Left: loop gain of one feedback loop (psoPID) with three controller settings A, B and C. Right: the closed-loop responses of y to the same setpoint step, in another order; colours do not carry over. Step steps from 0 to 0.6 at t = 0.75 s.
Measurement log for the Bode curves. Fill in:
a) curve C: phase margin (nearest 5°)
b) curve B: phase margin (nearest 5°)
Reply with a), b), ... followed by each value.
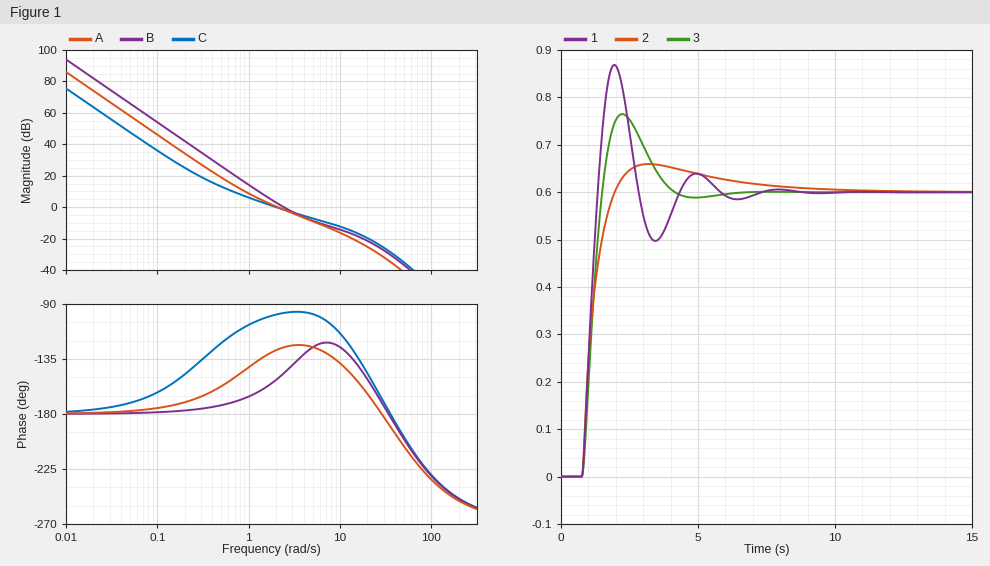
a) 80°
b) 35°
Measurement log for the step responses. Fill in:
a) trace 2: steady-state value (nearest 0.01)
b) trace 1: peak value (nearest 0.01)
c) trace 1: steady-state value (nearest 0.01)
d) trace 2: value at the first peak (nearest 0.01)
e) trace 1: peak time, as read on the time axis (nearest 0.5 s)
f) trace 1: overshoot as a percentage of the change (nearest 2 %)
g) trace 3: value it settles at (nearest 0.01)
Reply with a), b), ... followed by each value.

a) 0.60
b) 0.87
c) 0.60
d) 0.66
e) 2.0 s
f) 44 %
g) 0.60
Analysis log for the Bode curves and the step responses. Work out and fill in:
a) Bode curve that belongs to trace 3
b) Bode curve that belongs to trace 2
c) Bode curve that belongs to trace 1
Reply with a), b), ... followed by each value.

a) A
b) C
c) B
